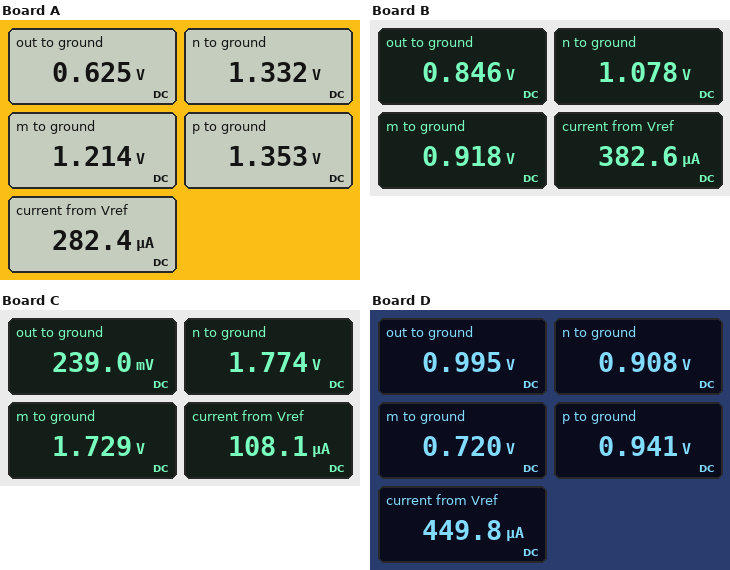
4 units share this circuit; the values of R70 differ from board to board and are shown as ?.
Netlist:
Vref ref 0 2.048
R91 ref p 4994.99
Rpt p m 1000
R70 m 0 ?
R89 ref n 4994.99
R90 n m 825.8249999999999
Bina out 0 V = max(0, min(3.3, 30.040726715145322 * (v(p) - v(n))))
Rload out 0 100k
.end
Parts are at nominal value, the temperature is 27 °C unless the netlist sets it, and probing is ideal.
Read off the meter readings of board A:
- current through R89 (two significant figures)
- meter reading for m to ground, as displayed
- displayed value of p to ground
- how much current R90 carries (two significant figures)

140 µA
1.214 V
1.353 V
140 µA
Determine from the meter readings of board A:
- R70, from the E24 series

4.3 kΩ
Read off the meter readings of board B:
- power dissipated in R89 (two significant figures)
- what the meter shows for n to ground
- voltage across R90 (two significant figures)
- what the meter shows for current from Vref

190 µW
1.078 V
160 mV
382.6 µA
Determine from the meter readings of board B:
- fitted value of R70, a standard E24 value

2.4 kΩ
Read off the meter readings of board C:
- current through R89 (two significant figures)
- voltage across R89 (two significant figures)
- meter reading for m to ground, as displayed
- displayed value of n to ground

55 µA
270 mV
1.729 V
1.774 V
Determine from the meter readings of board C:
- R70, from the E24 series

16 kΩ
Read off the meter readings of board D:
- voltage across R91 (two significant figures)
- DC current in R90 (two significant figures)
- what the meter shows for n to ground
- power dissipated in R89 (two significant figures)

1.1 V
230 µA
0.908 V
260 µW
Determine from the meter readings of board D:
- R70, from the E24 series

1.6 kΩ
